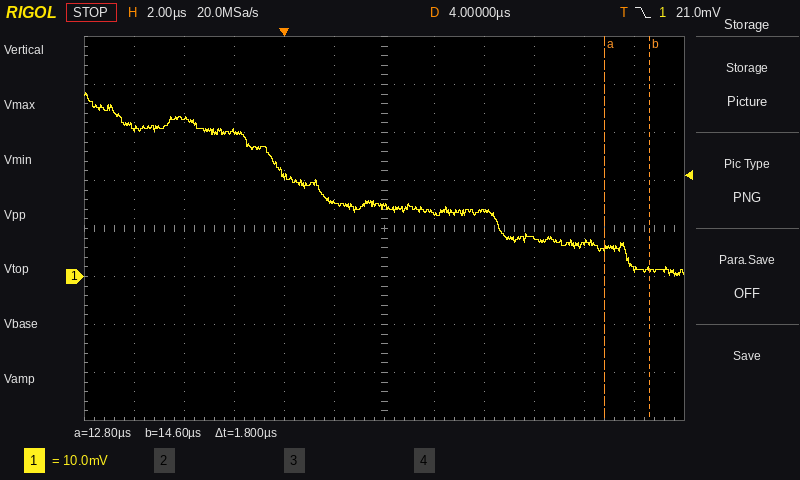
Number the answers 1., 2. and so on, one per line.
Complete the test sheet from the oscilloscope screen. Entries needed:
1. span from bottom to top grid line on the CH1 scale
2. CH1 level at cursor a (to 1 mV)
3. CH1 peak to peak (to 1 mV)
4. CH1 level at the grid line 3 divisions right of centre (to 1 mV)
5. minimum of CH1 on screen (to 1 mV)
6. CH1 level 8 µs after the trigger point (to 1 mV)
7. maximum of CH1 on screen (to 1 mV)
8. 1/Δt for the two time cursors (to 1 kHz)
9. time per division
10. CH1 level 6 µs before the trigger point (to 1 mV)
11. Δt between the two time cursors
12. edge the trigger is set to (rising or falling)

1. 80 mV
2. 6 mV
3. 38 mV
4. 8 mV
5. 0 mV
6. 14 mV
7. 38 mV
8. 556 kHz
9. 2 µs
10. 31 mV
11. 1.8 µs
12. falling
